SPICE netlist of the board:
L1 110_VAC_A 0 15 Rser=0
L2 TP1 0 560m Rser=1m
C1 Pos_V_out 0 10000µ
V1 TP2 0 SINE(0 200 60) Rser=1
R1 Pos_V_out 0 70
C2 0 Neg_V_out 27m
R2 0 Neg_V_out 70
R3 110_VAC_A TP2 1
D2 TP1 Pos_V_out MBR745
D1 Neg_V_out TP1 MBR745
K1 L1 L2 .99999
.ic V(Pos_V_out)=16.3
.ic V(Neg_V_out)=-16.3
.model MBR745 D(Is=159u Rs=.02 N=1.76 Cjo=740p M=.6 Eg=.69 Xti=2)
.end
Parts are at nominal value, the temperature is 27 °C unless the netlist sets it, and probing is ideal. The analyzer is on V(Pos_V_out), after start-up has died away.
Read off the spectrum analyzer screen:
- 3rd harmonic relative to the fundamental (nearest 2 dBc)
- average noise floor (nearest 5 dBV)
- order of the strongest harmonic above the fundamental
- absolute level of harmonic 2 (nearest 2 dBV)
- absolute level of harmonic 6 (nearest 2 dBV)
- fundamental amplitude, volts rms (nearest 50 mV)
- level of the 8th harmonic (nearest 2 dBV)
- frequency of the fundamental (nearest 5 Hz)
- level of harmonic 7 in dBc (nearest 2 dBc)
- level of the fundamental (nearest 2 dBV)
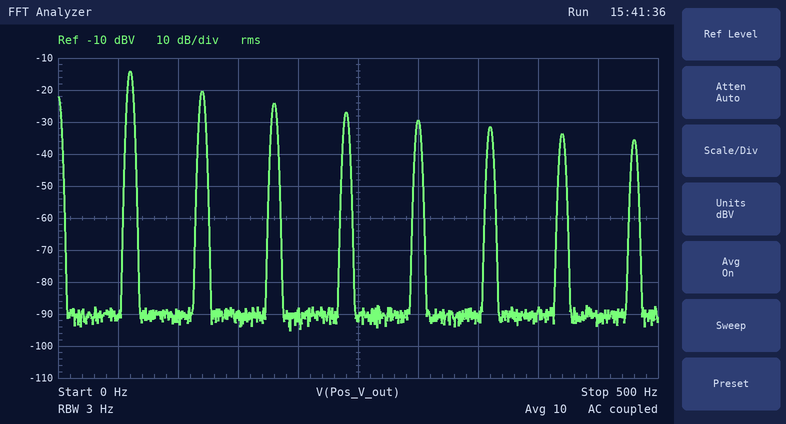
-10 dBc
-90 dBV
2
-20 dBV
-32 dBV
200 mV
-36 dBV
60 Hz
-20 dBc
-14 dBV
